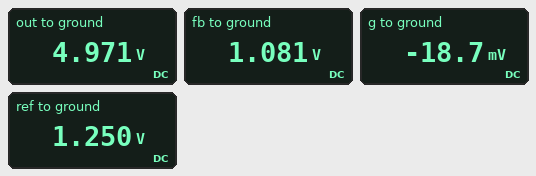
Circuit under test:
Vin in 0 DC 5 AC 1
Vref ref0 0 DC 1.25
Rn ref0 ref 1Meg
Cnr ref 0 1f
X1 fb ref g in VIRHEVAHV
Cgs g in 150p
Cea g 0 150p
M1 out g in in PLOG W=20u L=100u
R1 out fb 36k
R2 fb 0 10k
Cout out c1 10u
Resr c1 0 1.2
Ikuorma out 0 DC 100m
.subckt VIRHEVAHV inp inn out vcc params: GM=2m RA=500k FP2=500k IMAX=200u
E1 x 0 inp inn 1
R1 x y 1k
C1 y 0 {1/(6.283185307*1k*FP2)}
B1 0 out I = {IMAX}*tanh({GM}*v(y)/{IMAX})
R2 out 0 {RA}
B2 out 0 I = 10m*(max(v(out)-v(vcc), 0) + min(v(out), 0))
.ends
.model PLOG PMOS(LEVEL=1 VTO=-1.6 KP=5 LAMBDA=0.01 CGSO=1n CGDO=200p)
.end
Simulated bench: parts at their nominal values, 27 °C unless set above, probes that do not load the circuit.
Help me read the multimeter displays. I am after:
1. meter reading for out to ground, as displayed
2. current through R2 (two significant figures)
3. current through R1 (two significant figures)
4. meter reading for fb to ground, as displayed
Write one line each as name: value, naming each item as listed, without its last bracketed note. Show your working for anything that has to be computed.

meter reading for out to ground, as displayed: 4.971 V
current through R2: (1.081 V) / 10 kΩ = 110 µA
current through R1: (4.971 V - 1.081 V) / 36 kΩ = 110 µA
meter reading for fb to ground, as displayed: 1.081 V
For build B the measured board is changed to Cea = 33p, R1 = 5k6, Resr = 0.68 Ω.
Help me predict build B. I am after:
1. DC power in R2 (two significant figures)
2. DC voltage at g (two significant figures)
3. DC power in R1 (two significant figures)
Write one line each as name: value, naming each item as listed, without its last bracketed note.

DC power in R2: 160 µW
DC voltage at g: 3.0 V
DC power in R1: 88 µW
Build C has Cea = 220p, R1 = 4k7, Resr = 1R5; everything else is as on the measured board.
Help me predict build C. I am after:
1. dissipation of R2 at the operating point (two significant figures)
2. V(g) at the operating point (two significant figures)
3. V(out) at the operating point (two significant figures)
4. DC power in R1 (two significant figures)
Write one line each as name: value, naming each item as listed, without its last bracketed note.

dissipation of R2 at the operating point: 160 µW
V(g) at the operating point: 3.0 V
V(out) at the operating point: 1.8 V
DC power in R1: 74 µW
